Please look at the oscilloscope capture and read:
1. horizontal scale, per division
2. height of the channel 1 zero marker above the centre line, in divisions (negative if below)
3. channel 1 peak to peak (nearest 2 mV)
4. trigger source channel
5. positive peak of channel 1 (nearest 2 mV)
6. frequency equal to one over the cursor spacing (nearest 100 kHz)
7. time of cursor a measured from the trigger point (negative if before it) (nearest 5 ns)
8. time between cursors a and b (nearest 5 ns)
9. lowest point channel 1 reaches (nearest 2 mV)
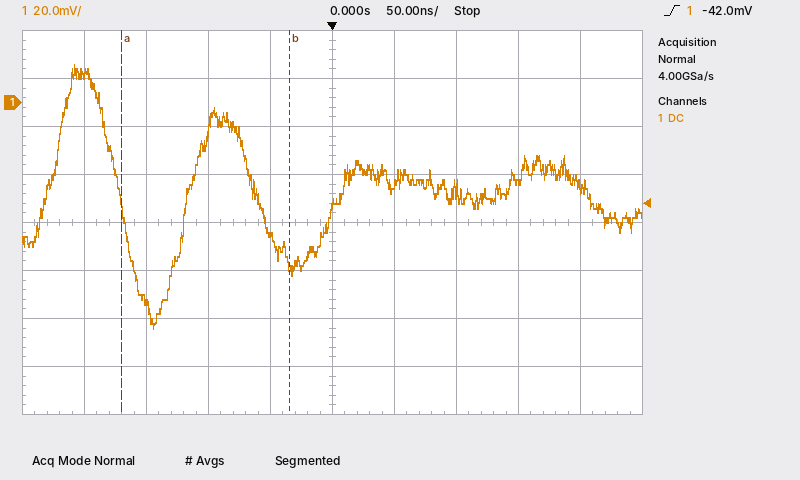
50 ns
+2.5 div
110 mV
channel 1
16 mV
7.4 MHz
-170 ns
135 ns
-94 mV
